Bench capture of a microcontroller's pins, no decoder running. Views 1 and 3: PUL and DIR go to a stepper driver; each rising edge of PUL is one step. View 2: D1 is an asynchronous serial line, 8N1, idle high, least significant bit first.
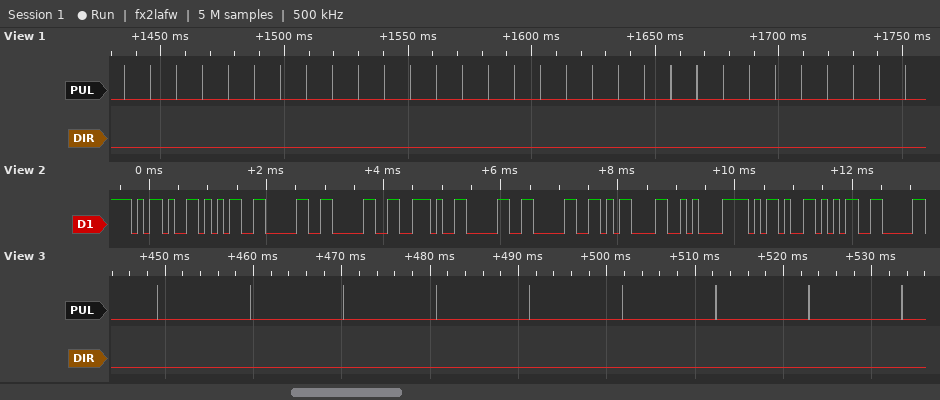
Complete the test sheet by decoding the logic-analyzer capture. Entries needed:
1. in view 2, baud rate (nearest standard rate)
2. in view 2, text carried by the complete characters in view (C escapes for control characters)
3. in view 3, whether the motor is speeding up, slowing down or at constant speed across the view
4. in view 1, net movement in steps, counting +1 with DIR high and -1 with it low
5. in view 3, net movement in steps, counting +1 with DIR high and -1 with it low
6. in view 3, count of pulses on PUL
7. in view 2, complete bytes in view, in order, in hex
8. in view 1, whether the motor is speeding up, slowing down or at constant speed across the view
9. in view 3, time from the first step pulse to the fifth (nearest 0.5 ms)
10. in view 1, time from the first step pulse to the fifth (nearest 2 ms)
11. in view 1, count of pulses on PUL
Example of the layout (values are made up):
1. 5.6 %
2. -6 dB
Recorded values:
1. 9600 baud
2. "-500.00\r\n-5"
3. constant speed
4. -31
5. -9
6. 9
7. 2D 35 30 30 2E 30 30 0D 0A 2D 35
8. constant speed
9. 42.0 ms
10. 42 ms
11. 31
